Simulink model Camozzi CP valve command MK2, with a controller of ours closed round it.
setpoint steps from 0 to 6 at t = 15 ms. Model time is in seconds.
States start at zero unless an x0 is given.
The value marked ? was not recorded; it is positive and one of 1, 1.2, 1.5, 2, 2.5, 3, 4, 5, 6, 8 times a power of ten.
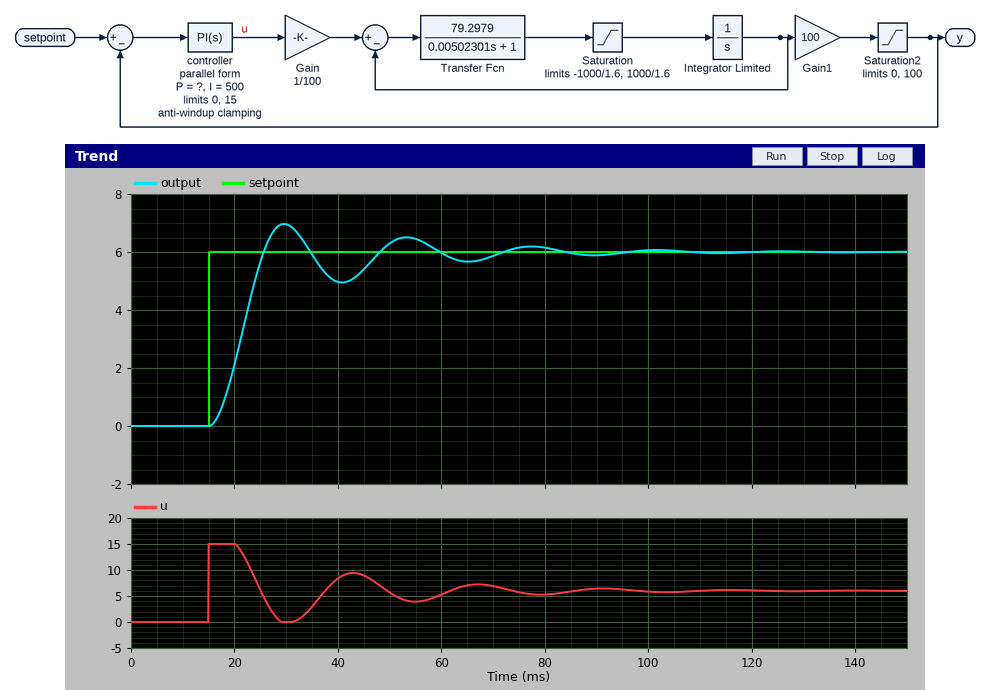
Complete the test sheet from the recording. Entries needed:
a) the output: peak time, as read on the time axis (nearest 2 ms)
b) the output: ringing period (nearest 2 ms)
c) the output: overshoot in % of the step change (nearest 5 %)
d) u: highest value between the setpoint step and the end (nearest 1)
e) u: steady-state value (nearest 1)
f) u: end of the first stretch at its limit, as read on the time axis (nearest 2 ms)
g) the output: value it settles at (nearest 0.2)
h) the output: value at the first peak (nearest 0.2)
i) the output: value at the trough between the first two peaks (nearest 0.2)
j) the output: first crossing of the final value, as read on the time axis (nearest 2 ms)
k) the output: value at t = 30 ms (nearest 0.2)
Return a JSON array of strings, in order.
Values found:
["30 ms", "24 ms", "15 %", "15", "6", "20 ms", "6.0", "7.0", "5.0", "26 ms", "7.0"]
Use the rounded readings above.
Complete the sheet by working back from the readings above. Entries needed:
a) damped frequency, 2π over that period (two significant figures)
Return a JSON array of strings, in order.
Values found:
["0.26 rad/ms"]
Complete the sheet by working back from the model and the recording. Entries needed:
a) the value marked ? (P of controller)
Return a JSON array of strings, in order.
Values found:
["4"]
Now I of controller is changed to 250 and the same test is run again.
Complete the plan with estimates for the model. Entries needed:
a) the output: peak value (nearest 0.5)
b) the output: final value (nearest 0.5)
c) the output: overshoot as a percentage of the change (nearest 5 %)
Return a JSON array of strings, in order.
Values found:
["6.5", "6.0", "10 %"]
